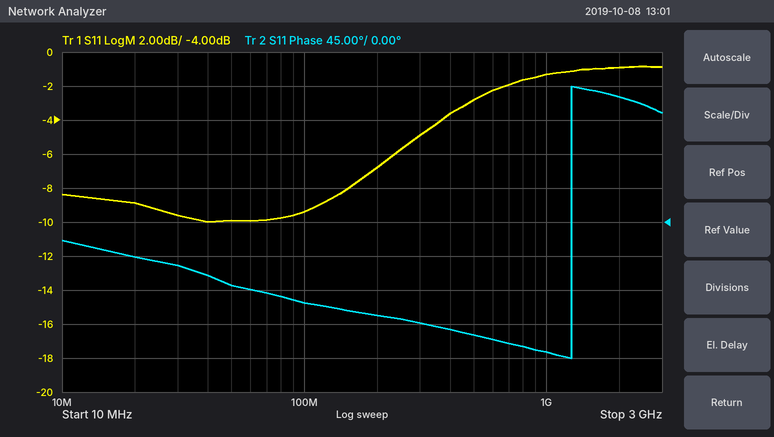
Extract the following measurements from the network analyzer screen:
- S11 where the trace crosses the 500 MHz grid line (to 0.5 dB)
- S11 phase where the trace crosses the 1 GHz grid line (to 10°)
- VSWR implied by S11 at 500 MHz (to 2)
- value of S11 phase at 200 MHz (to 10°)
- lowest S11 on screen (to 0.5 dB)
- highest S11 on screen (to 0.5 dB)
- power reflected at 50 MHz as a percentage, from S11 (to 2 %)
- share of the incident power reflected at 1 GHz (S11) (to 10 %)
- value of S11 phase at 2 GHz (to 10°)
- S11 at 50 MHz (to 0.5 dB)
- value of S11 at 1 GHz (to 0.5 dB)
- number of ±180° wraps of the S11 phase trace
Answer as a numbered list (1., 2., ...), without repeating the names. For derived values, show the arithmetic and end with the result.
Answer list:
1. -3.0 dB
2. -170°
3. |Γ| = 10^(-3/20) = 0.7079; VSWR = (1 + 0.7079)/(1 − 0.7079) ≈ 6
4. -120°
5. -10.0 dB
6. -1.0 dB
7. 10^(-10/10) ≈ 10 %
8. 10^(-1.5/10) ≈ 70.8 %, so 70 % to the nearest 10 %
9. 170°
10. -10.0 dB
11. -1.5 dB
12. 1
